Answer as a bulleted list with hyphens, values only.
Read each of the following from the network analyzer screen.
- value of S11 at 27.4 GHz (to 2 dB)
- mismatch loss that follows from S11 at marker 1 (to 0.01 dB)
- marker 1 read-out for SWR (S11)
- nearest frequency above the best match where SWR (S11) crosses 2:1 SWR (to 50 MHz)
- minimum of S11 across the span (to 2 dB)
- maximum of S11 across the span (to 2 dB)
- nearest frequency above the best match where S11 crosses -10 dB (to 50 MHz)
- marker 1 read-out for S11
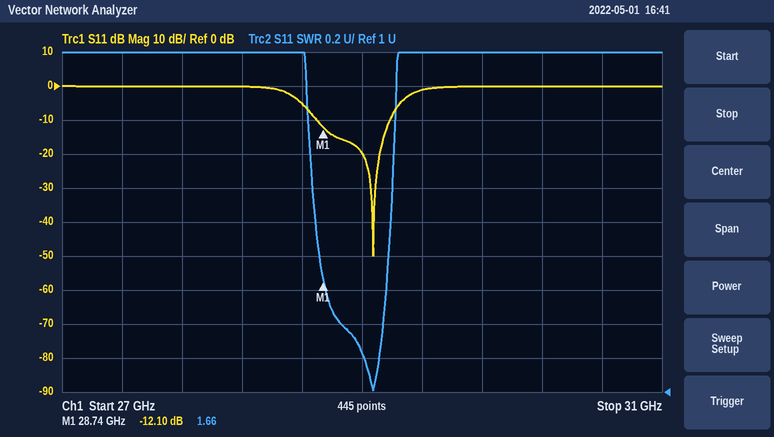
- 0 dB
- 0.28 dB
- 1.66
- 29.20 GHz
- -50 dB
- 0 dB
- 29.20 GHz
- -12.10 dB
